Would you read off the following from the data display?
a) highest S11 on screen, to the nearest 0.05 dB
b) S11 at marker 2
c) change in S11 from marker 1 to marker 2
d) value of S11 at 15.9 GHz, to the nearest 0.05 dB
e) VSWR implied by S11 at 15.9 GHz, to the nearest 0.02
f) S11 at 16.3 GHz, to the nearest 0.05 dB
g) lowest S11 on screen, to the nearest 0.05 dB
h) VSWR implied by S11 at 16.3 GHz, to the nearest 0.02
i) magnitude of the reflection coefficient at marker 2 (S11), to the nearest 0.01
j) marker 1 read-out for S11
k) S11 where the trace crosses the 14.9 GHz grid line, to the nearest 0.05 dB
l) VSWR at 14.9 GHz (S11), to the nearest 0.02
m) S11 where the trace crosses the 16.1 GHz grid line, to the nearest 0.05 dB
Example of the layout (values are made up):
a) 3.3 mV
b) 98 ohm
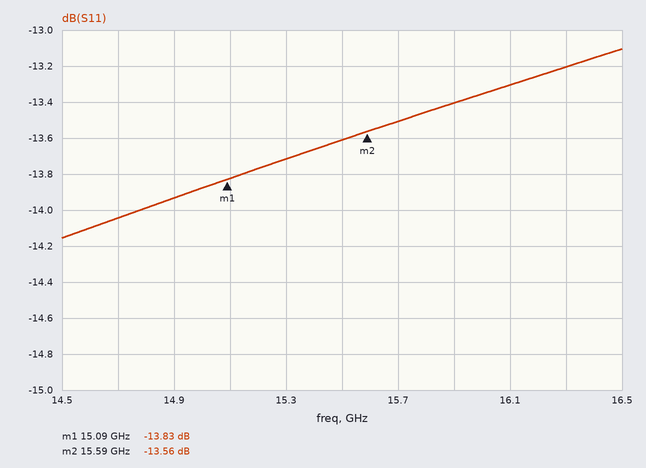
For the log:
a) -13.10 dB
b) -13.56 dB
c) 0.27 dB
d) -13.40 dB
e) 1.54
f) -13.20 dB
g) -14.15 dB
h) 1.56
i) 0.21
j) -13.83 dB
k) -13.95 dB
l) 1.50
m) -13.30 dB
